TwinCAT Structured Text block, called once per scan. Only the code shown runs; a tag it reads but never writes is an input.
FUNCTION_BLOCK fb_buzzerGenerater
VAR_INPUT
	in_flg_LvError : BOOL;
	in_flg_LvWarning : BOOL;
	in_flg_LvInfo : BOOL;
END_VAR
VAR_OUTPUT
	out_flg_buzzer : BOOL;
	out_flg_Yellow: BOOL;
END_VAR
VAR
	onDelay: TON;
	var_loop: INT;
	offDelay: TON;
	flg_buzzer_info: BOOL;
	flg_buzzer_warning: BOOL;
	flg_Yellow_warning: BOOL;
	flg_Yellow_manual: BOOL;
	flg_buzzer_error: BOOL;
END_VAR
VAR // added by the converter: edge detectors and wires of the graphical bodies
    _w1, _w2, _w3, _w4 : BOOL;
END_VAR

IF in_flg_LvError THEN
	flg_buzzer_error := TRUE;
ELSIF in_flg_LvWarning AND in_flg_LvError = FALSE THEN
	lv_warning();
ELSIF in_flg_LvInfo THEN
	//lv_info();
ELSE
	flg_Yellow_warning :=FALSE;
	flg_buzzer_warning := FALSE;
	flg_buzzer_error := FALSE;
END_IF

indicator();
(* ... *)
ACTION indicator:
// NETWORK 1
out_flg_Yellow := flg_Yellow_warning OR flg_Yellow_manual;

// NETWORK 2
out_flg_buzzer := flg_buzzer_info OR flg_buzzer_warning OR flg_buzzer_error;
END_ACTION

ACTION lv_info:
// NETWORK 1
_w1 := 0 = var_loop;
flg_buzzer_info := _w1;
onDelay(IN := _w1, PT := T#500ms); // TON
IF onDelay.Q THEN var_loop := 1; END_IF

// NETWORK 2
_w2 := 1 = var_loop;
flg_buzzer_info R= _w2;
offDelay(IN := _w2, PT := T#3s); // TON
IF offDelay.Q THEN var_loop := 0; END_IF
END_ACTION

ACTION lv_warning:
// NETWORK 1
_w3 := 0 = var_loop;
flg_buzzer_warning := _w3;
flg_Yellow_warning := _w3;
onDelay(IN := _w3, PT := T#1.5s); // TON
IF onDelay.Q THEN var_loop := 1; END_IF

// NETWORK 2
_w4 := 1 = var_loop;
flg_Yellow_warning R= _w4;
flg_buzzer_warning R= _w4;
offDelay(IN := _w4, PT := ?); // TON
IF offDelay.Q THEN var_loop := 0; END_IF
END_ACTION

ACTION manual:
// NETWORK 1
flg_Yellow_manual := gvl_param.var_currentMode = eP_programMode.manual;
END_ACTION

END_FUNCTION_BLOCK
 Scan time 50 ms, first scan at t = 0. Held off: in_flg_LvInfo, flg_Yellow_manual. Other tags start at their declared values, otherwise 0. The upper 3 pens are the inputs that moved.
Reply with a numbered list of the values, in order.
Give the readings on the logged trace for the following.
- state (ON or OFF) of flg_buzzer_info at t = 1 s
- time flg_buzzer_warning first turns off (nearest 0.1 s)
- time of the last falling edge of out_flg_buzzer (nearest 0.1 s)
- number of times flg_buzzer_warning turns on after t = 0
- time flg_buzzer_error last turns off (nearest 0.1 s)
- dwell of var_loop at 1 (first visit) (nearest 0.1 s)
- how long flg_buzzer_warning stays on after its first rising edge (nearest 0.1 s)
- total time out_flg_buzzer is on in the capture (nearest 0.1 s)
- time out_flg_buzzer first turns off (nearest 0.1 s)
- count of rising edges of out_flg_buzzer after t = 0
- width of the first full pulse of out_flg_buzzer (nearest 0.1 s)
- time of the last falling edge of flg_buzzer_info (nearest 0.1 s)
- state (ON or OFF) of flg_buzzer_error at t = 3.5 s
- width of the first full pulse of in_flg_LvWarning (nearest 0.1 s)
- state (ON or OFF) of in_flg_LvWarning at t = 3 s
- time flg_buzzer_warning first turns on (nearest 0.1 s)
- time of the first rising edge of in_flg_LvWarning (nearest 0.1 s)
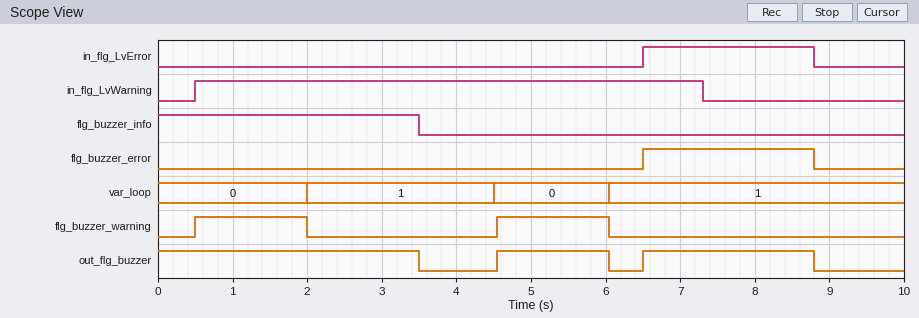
1. ON
2. 2.0 s
3. 8.8 s
4. 2
5. 8.8 s
6. 2.5 s
7. 1.5 s
8. 7.3 s
9. 3.5 s
10. 2
11. 1.5 s
12. 3.5 s
13. OFF
14. 6.8 s
15. ON
16. 0.5 s
17. 0.5 s
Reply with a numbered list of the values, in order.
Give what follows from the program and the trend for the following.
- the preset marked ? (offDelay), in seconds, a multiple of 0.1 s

1. 2.5 s
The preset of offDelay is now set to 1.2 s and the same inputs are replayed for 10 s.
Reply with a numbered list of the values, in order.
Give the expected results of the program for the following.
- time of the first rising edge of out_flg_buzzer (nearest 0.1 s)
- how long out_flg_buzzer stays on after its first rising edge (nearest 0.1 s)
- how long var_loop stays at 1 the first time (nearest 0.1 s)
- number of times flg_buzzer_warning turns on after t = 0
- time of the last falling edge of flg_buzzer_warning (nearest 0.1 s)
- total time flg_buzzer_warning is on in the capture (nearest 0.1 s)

1. 6.0 s
2. 2.8 s
3. 1.2 s
4. 3
5. 8.8 s
6. 5.8 s
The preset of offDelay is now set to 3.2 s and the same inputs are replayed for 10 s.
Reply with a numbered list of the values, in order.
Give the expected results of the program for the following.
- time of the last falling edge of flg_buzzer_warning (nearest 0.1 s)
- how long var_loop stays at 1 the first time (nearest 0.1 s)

1. 8.8 s
2. 3.2 s
